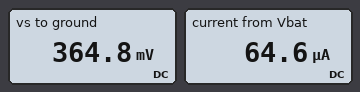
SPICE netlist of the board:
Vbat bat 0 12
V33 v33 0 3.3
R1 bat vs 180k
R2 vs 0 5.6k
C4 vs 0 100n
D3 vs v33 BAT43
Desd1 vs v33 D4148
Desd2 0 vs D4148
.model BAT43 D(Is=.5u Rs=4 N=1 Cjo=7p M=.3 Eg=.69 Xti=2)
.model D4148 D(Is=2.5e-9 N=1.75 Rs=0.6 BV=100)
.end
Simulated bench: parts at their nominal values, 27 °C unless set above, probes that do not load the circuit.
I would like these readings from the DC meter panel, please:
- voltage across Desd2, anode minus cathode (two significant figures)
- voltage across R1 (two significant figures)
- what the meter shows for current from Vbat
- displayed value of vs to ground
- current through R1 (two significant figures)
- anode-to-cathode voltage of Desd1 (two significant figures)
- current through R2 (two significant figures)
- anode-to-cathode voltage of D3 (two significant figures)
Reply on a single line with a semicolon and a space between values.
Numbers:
-360 mV; 12 V; 64.6 µA; 364.8 mV; 65 µA; -2.9 V; 65 µA; -2.9 V
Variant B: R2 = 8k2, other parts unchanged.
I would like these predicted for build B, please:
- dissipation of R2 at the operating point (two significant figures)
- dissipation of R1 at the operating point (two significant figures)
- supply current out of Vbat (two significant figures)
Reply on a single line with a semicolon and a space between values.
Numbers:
34 µW; 730 µW; 64 µA
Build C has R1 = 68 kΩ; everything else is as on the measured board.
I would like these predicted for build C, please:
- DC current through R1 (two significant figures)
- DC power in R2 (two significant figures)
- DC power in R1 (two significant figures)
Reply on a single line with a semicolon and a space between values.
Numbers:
160 µA; 150 µW; 1.8 mW
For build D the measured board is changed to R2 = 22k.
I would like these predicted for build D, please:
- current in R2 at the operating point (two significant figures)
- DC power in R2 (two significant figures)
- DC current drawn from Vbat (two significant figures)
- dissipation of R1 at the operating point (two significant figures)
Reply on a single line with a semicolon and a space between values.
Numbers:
60 µA; 79 µW; 59 µA; 630 µW
